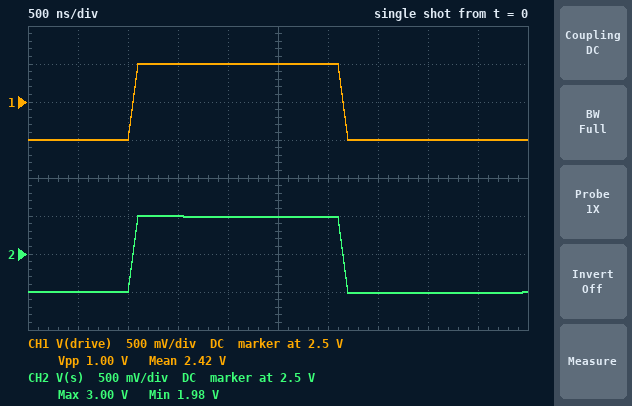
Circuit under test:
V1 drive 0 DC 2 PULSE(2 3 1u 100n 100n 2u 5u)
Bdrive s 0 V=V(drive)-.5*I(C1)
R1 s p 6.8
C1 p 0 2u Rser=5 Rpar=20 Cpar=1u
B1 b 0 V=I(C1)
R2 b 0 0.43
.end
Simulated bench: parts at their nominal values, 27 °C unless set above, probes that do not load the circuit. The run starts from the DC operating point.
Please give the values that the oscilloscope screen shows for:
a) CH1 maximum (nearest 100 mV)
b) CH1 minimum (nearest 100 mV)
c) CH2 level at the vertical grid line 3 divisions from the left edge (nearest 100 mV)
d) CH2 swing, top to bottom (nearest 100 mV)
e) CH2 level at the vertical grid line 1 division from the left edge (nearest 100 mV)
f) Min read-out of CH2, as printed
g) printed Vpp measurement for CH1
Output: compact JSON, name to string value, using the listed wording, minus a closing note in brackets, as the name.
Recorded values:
{"CH1 maximum": "3.0 V", "CH1 minimum": "2.0 V", "CH2 level at the vertical grid line 3 divisions from the left edge": "3.0 V", "CH2 swing, top to bottom": "1.0 V", "CH2 level at the vertical grid line 1 division from the left edge": "2.0 V", "Min read-out of CH2, as printed": "1.98 V", "printed Vpp measurement for CH1": "1.00 V"}
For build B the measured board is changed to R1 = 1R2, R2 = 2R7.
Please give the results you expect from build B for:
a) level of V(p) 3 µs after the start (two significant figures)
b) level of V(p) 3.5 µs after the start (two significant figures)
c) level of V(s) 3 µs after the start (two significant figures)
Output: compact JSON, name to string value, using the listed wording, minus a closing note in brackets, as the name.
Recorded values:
{"level of V(p) 3 µs after the start": "2.5 V", "level of V(p) 3.5 µs after the start": "2.3 V", "level of V(s) 3 µs after the start": "2.9 V"}
